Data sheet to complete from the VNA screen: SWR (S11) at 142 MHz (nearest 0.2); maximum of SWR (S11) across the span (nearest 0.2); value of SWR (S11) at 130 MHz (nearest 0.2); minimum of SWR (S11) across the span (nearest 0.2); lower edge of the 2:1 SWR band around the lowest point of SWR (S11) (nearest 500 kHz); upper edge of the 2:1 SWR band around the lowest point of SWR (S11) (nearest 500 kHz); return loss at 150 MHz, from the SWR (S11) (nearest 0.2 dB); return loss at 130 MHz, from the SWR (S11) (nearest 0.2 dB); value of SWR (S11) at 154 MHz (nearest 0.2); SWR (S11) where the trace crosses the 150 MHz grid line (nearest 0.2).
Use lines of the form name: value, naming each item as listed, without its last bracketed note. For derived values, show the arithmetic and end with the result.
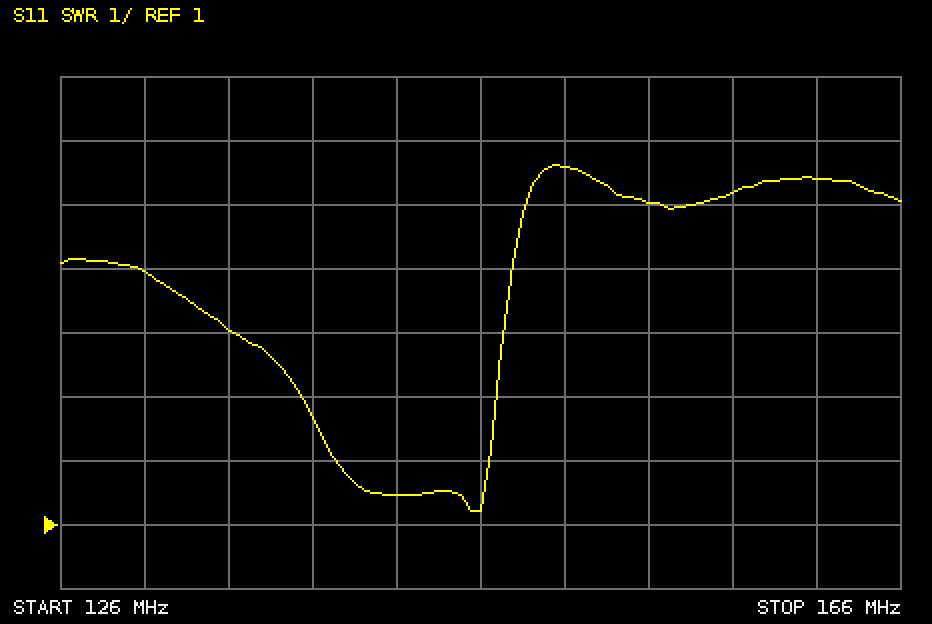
SWR (S11) at 142 MHz: 1.4
maximum of SWR (S11) across the span: 6.6
value of SWR (S11) at 130 MHz: 5.0
minimum of SWR (S11) across the span: 1.2
lower edge of the 2:1 SWR band around the lowest point of SWR (S11): 139.0 MHz
upper edge of the 2:1 SWR band around the lowest point of SWR (S11): 146.5 MHz
return loss at 150 MHz, from the SWR (S11): −20 log10((6.6 − 1)/(6.6 + 1)) ≈ 2.6 dB
return loss at 130 MHz, from the SWR (S11): −20 log10((5 − 1)/(5 + 1)) ≈ 3.52 dB, so 3.6 dB to the nearest 0.2 dB
value of SWR (S11) at 154 MHz: 6.0
SWR (S11) where the trace crosses the 150 MHz grid line: 6.6
